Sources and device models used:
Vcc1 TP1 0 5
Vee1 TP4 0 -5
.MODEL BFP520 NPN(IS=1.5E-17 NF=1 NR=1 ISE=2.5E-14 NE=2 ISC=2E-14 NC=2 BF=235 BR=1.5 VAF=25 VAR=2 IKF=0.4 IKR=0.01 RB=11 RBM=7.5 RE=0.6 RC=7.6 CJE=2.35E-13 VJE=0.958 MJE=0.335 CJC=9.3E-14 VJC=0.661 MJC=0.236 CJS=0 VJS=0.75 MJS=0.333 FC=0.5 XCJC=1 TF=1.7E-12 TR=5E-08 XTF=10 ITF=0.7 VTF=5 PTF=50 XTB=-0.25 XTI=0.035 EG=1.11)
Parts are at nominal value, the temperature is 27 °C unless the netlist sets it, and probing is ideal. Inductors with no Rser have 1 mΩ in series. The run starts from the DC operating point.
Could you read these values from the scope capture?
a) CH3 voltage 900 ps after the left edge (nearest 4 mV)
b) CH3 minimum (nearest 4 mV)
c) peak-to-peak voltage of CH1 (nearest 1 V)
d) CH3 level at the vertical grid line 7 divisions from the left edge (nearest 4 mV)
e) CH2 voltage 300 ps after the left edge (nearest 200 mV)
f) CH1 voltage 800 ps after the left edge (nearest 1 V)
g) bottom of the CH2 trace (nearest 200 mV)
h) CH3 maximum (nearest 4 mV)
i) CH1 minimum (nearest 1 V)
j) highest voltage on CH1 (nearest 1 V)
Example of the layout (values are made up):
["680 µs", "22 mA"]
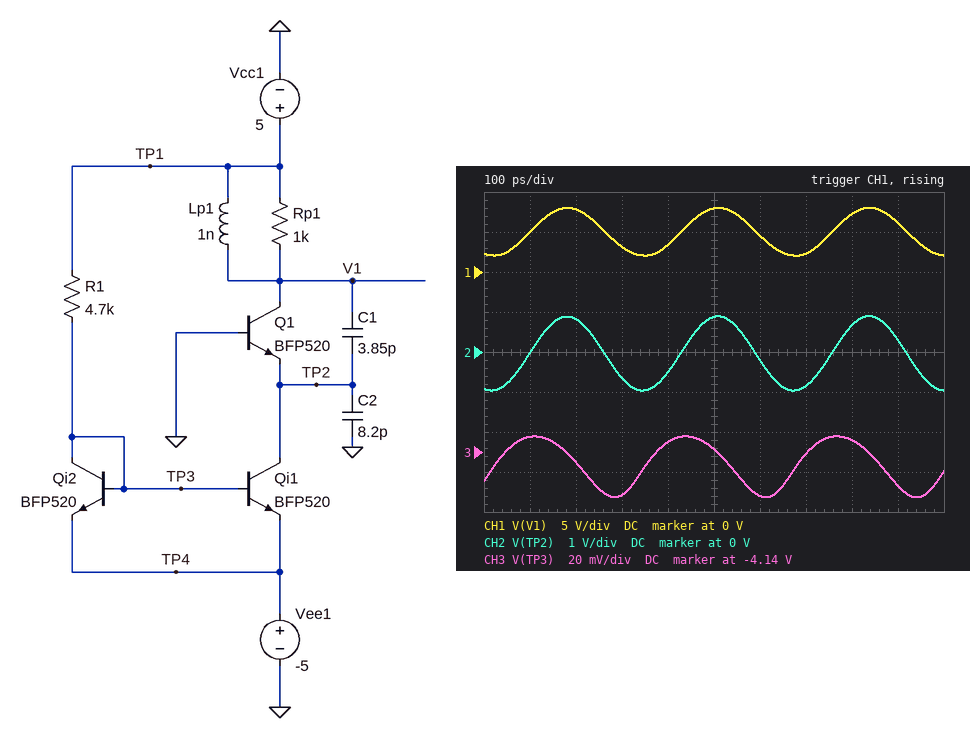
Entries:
["-4.156 V", "-4.164 V", "6 V", "-4.140 V", "-600 mV", "7 V", "-1.0 V", "-4.132 V", "2 V", "8 V"]
